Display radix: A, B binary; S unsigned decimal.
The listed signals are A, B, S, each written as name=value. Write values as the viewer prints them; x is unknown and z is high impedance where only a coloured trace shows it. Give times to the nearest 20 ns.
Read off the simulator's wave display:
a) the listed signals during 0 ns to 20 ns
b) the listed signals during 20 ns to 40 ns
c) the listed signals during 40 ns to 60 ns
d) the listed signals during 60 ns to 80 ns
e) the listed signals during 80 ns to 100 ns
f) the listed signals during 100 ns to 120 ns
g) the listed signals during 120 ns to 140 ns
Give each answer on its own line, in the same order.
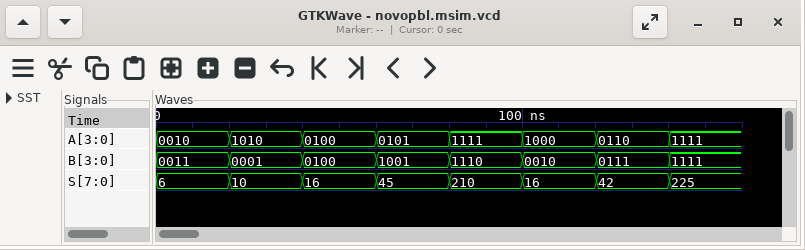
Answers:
A=0010, B=0011, S=6
A=1010, B=0001, S=10
A=0100, B=0100, S=16
A=0101, B=1001, S=45
A=1111, B=1110, S=210
A=1000, B=0010, S=16
A=0110, B=0111, S=42
